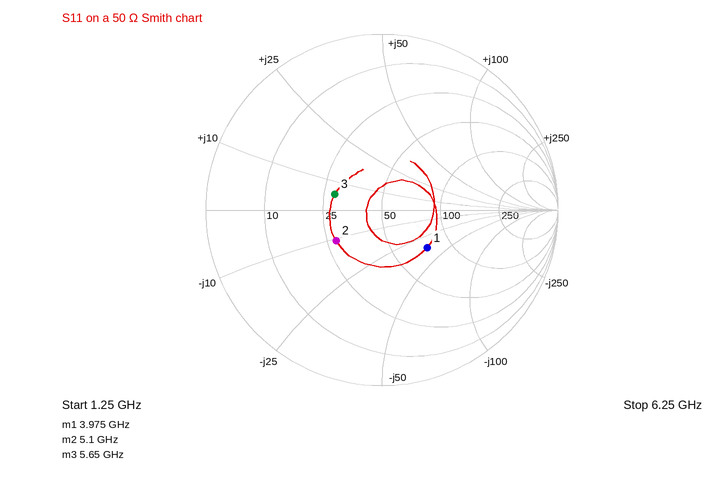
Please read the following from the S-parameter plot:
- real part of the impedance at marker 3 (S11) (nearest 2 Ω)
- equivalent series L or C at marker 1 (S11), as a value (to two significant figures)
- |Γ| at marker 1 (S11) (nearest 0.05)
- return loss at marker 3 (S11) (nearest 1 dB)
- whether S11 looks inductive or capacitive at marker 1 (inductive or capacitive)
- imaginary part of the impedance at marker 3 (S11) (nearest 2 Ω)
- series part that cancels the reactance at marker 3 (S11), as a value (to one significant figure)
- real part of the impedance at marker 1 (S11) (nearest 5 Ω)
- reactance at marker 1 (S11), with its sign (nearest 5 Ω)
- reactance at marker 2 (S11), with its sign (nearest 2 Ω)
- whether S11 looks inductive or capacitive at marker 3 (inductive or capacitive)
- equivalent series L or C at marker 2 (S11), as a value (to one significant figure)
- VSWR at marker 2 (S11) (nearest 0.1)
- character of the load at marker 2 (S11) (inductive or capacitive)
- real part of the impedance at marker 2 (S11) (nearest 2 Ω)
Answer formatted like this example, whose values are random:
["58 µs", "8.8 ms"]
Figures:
["28 Ω", "1.1 pF", "0.35", "11 dB", "capacitive", "+6 Ω", "5 pF", "75 Ω", "-35 Ω", "-10 Ω", "inductive", "3 pF", "1.9", "capacitive", "28 Ω"]
